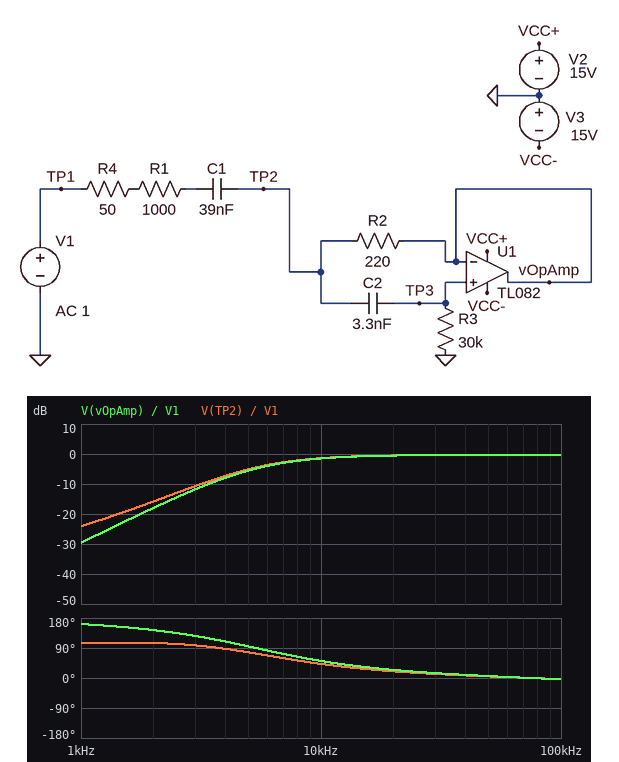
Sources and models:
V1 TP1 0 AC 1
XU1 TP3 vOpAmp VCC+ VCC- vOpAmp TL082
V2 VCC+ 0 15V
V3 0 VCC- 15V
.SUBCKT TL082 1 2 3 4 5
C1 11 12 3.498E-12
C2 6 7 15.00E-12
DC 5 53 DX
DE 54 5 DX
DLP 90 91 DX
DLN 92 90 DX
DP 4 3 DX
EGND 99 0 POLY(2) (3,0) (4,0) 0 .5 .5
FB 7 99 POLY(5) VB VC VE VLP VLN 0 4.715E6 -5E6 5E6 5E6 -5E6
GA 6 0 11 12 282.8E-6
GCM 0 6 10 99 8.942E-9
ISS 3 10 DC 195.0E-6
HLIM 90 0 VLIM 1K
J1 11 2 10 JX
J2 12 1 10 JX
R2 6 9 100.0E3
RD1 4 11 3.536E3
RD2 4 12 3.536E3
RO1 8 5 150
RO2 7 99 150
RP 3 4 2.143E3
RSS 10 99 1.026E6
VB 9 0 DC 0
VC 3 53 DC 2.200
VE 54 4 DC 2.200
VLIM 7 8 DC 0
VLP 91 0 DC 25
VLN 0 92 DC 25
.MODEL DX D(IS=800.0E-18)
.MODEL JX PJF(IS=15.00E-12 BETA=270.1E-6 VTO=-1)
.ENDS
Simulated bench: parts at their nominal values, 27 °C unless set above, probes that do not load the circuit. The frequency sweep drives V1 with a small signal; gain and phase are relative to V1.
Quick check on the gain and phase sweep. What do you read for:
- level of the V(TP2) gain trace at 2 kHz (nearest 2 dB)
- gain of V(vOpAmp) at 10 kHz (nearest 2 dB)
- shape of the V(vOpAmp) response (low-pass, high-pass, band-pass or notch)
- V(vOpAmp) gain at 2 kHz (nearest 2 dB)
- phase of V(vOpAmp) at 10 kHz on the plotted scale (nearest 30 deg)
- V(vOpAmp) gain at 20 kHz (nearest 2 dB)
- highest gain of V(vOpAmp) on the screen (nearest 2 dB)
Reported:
-16 dB
-2 dB
high-pass
-18 dB
60 deg
0 dB
0 dB
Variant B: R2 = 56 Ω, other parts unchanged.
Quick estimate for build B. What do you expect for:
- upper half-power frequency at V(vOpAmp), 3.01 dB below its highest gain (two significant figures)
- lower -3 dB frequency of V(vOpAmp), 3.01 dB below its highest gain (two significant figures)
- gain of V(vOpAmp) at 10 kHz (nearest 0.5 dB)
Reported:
190 kHz
24 kHz
-10.0 dB
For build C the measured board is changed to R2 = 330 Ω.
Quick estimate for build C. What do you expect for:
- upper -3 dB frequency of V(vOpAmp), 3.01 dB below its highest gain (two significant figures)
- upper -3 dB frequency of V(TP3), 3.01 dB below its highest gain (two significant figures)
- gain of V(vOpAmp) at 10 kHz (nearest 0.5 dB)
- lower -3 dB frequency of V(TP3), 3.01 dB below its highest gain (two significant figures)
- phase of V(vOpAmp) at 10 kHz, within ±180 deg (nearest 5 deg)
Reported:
850 kHz
900 kHz
-0.5 dB
4.7 kHz
40 deg
